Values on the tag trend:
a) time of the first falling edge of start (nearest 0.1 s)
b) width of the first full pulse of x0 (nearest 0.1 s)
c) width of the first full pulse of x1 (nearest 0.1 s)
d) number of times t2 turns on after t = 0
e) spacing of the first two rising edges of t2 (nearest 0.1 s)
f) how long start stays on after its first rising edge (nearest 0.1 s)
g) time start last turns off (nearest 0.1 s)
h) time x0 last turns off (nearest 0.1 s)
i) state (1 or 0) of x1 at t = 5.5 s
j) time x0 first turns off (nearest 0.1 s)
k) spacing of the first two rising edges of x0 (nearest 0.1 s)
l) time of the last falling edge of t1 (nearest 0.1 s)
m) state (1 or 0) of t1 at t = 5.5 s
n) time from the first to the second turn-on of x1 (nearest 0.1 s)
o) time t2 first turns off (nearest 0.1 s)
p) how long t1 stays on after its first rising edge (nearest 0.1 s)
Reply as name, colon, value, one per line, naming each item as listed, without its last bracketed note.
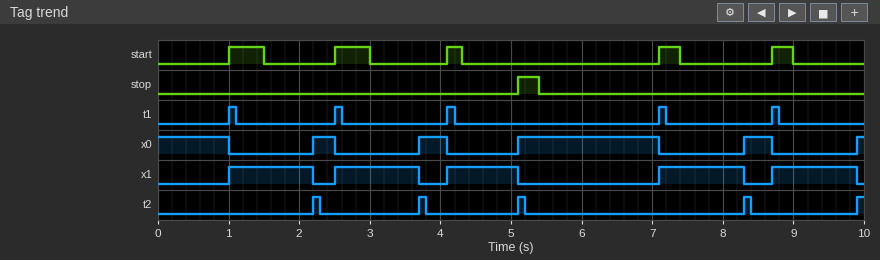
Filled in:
time of the first falling edge of start: 1.5 s
width of the first full pulse of x0: 0.3 s
width of the first full pulse of x1: 1.2 s
number of times t2 turns on after t = 0: 5
spacing of the first two rising edges of t2: 1.5 s
how long start stays on after its first rising edge: 0.5 s
time start last turns off: 9.0 s
time x0 last turns off: 8.7 s
state (1 or 0) of x1 at t = 5.5 s: 0
time x0 first turns off: 1.0 s
spacing of the first two rising edges of x0: 1.5 s
time of the last falling edge of t1: 8.8 s
state (1 or 0) of t1 at t = 5.5 s: 0
time from the first to the second turn-on of x1: 1.5 s
time t2 first turns off: 2.3 s
how long t1 stays on after its first rising edge: 0.1 s
